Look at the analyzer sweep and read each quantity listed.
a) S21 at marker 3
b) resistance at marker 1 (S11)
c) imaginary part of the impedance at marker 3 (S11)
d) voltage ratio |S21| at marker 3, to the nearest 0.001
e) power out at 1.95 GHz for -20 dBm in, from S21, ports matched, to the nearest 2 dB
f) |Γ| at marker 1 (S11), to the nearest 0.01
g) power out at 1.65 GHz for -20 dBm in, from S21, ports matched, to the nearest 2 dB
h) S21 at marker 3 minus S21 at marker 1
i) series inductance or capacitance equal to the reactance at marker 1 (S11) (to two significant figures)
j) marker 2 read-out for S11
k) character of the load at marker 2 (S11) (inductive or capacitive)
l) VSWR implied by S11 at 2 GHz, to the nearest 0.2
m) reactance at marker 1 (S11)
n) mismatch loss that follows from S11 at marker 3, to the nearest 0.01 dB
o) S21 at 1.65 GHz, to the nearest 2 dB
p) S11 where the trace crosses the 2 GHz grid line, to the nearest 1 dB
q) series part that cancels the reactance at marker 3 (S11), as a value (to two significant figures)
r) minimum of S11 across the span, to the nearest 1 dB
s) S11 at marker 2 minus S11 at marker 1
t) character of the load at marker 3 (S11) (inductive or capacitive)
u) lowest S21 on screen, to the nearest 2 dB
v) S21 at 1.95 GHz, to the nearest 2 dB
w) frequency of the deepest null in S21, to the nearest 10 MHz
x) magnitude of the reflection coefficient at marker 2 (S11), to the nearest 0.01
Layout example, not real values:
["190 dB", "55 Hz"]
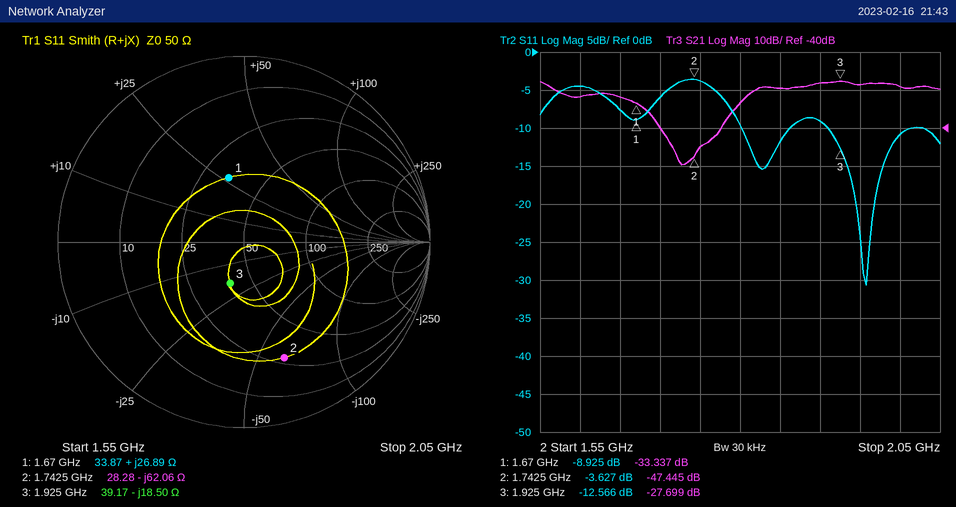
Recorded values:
["-27.699 dB", "33.87 Ω", "-18.50 Ω", "0.041", "-48 dBm", "0.36", "-52 dBm", "5.638 dB", "2.6 nH", "-3.627 dB", "capacitive", "1.8", "+26.89 Ω", "0.25 dB", "-32 dB", "-11 dB", "1.5 nH", "-31 dB", "5.298 dB", "capacitive", "-50 dB", "-28 dB", "1.73 GHz", "0.66"]
